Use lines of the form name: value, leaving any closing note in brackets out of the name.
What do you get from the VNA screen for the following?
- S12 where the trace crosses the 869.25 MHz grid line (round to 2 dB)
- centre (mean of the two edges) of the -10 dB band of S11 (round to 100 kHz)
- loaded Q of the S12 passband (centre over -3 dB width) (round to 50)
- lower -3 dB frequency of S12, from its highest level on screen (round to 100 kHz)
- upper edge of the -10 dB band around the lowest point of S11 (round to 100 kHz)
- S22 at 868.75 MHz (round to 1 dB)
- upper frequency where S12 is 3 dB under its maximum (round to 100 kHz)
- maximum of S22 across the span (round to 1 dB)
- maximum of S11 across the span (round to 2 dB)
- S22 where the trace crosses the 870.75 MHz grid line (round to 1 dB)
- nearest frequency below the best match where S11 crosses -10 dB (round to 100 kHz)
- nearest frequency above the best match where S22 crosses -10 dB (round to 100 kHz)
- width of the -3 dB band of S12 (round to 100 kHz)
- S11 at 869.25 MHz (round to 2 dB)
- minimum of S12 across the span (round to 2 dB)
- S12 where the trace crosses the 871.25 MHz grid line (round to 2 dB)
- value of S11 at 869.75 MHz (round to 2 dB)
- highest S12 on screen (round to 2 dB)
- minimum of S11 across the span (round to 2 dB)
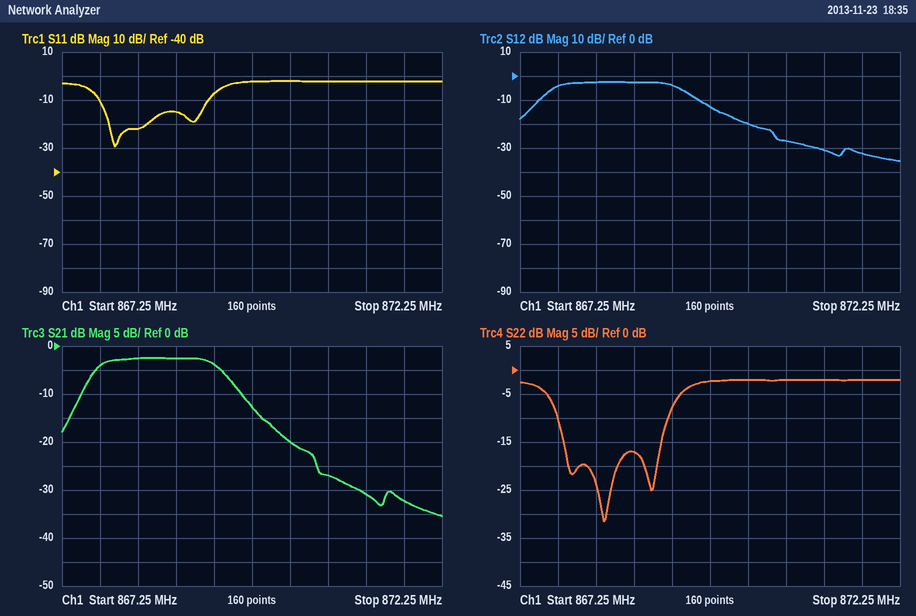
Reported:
S12 where the trace crosses the 869.25 MHz grid line: -4 dB
centre (mean of the two edges) of the -10 dB band of S11: 868.5 MHz
loaded Q of the S12 passband (centre over -3 dB width): 500
lower -3 dB frequency of S12, from its highest level on screen: 867.7 MHz
upper edge of the -10 dB band around the lowest point of S11: 869.2 MHz
S22 at 868.75 MHz: -17 dB
upper frequency where S12 is 3 dB under its maximum: 869.4 MHz
maximum of S22 across the span: -2 dB
maximum of S11 across the span: -2 dB
S22 where the trace crosses the 870.75 MHz grid line: -2 dB
nearest frequency below the best match where S11 crosses -10 dB: 867.7 MHz
nearest frequency above the best match where S22 crosses -10 dB: 869.2 MHz
width of the -3 dB band of S12: 1.7 MHz
S11 at 869.25 MHz: -8 dB
minimum of S12 across the span: -36 dB
S12 where the trace crosses the 871.25 MHz grid line: -30 dB
value of S11 at 869.75 MHz: -2 dB
highest S12 on screen: -2 dB
minimum of S11 across the span: -30 dB
